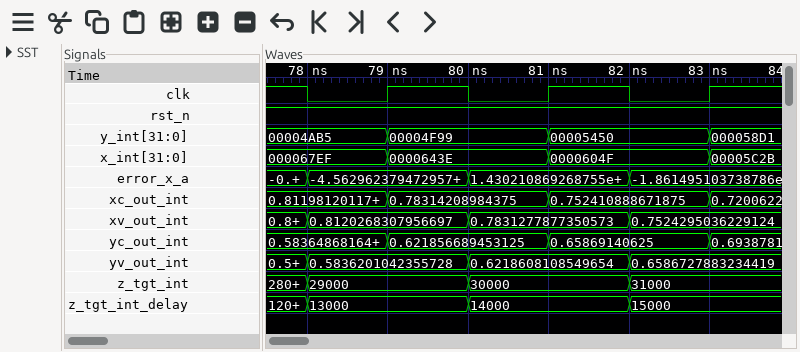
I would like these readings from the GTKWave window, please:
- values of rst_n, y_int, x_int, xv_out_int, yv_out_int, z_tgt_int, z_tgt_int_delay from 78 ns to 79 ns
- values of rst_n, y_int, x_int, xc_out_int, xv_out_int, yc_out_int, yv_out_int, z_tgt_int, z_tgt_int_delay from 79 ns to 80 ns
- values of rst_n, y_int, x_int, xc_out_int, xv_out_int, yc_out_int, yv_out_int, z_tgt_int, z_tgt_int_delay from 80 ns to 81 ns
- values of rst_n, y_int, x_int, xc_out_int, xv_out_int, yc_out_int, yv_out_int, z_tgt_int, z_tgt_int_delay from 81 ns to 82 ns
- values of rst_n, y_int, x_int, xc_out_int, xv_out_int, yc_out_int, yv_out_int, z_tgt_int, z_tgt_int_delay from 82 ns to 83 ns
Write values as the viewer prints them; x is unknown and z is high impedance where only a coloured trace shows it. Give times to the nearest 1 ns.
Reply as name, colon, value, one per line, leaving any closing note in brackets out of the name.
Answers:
values of rst_n, y_int, x_int, xv_out_int, yv_out_int, z_tgt_int, z_tgt_int_delay from 78 ns to 79 ns: rst_n=1, y_int=00004AB5, x_int=000067EF, xv_out_int=0.8120268307956697, yv_out_int=0.5836201042355728, z_tgt_int=29000, z_tgt_int_delay=13000
values of rst_n, y_int, x_int, xc_out_int, xv_out_int, yc_out_int, yv_out_int, z_tgt_int, z_tgt_int_delay from 79 ns to 80 ns: rst_n=1, y_int=00004F99, x_int=0000643E, xc_out_int=0.78314208984375, xv_out_int=0.8120268307956697, yc_out_int=0.621856689453125, yv_out_int=0.5836201042355728, z_tgt_int=29000, z_tgt_int_delay=13000
values of rst_n, y_int, x_int, xc_out_int, xv_out_int, yc_out_int, yv_out_int, z_tgt_int, z_tgt_int_delay from 80 ns to 81 ns: rst_n=1, y_int=00004F99, x_int=0000643E, xc_out_int=0.78314208984375, xv_out_int=0.7831277877350573, yc_out_int=0.621856689453125, yv_out_int=0.6218608108549654, z_tgt_int=30000, z_tgt_int_delay=14000
values of rst_n, y_int, x_int, xc_out_int, xv_out_int, yc_out_int, yv_out_int, z_tgt_int, z_tgt_int_delay from 81 ns to 82 ns: rst_n=1, y_int=00005450, x_int=0000604F, xc_out_int=0.752410888671875, xv_out_int=0.7831277877350573, yc_out_int=0.65869140625, yv_out_int=0.6218608108549654, z_tgt_int=30000, z_tgt_int_delay=14000
values of rst_n, y_int, x_int, xc_out_int, xv_out_int, yc_out_int, yv_out_int, z_tgt_int, z_tgt_int_delay from 82 ns to 83 ns: rst_n=1, y_int=00005450, x_int=0000604F, xc_out_int=0.752410888671875, xv_out_int=0.7524295036229124, yc_out_int=0.65869140625, yv_out_int=0.6586727883234419, z_tgt_int=31000, z_tgt_int_delay=15000
